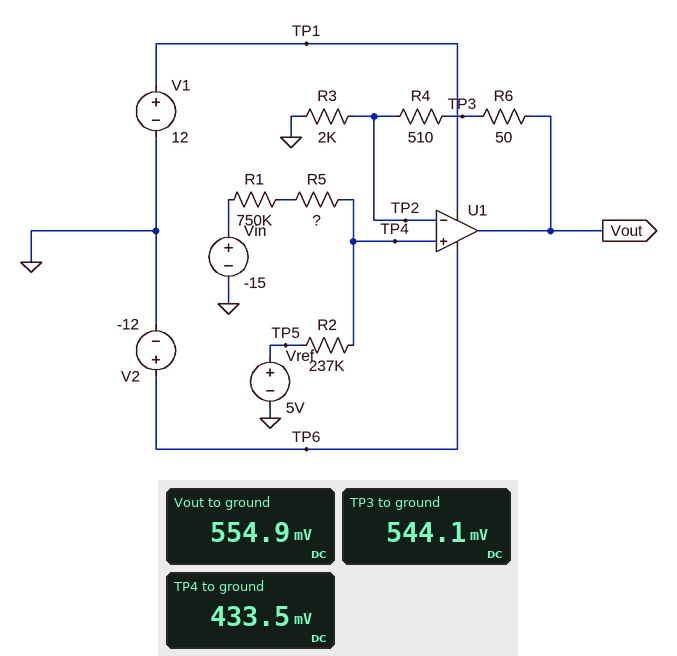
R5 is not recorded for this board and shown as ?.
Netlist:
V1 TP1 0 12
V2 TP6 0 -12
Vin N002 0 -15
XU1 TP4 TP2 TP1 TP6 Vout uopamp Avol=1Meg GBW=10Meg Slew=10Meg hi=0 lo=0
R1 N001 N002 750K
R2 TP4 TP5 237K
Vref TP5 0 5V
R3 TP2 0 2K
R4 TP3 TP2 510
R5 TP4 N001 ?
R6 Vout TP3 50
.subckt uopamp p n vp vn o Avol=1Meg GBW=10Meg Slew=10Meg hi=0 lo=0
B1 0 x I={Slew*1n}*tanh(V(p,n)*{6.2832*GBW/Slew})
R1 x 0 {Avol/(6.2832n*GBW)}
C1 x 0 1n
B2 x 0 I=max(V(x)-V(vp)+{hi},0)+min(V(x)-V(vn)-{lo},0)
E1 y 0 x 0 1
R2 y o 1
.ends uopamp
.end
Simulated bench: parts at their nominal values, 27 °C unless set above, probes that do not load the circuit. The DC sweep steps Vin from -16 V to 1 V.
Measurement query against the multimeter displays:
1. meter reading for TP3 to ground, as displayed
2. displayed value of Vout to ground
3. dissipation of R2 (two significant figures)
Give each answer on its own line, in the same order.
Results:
544.1 mV
554.9 mV
88 µW
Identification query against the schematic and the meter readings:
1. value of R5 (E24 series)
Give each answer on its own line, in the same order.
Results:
51 kΩ
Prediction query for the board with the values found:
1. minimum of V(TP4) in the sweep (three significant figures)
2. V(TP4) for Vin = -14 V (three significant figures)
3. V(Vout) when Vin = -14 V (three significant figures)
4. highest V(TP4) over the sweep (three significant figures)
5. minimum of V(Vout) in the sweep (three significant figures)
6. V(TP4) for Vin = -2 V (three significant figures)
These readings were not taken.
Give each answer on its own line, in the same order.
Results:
205 mV
662 mV
847 mV
4.09 V
263 mV
3.40 V
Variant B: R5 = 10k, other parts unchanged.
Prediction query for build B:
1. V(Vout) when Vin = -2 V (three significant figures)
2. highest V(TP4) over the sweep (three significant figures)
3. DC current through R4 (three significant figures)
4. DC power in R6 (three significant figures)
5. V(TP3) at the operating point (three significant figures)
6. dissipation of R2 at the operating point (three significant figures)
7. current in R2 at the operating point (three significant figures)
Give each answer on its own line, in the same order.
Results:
4.27 V
4.05 V
123 µA
755 nW
308 mV
95.4 µW
20.1 µA
